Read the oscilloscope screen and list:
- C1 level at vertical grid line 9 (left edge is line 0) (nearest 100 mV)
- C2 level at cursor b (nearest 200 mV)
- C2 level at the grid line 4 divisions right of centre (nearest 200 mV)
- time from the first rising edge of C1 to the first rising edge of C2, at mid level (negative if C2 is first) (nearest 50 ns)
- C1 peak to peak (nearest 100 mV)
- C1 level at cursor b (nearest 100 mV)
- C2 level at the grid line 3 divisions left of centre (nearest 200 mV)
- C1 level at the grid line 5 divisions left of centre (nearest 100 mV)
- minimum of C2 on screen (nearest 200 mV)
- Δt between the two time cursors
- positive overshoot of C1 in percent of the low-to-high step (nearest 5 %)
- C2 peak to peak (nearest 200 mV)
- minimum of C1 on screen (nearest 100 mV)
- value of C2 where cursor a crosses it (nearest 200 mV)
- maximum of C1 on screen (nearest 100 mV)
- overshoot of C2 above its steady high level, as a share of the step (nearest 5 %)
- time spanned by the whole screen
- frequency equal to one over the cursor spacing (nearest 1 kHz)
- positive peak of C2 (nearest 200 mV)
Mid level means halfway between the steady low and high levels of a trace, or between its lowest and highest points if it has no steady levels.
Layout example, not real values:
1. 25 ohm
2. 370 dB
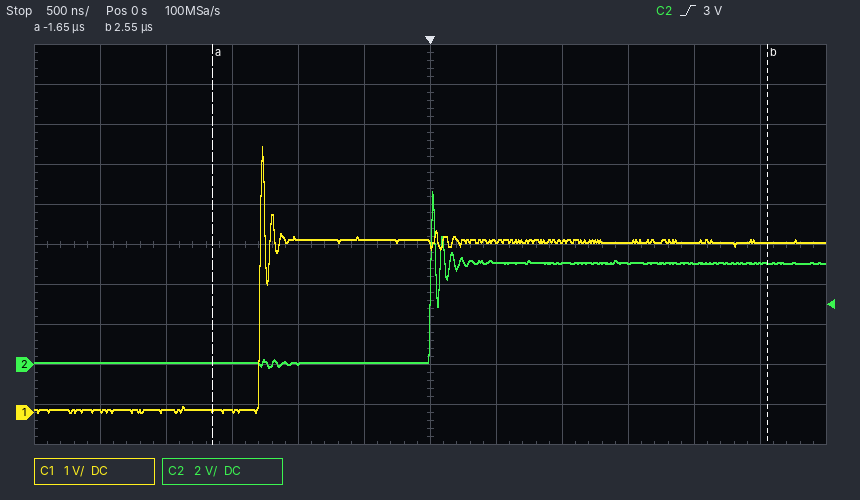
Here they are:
1. 4.2 V
2. 5.0 V
3. 5.0 V
4. +1.30 µs
5. 6.6 V
6. 4.2 V
7. 0.0 V
8. 0.0 V
9. -200 mV
10. 4.20 µs
11. 55 %
12. 8.8 V
13. 0.0 V
14. 0.0 V
15. 6.6 V
16. 70 %
17. 6 µs
18. 238 kHz
19. 8.6 V
